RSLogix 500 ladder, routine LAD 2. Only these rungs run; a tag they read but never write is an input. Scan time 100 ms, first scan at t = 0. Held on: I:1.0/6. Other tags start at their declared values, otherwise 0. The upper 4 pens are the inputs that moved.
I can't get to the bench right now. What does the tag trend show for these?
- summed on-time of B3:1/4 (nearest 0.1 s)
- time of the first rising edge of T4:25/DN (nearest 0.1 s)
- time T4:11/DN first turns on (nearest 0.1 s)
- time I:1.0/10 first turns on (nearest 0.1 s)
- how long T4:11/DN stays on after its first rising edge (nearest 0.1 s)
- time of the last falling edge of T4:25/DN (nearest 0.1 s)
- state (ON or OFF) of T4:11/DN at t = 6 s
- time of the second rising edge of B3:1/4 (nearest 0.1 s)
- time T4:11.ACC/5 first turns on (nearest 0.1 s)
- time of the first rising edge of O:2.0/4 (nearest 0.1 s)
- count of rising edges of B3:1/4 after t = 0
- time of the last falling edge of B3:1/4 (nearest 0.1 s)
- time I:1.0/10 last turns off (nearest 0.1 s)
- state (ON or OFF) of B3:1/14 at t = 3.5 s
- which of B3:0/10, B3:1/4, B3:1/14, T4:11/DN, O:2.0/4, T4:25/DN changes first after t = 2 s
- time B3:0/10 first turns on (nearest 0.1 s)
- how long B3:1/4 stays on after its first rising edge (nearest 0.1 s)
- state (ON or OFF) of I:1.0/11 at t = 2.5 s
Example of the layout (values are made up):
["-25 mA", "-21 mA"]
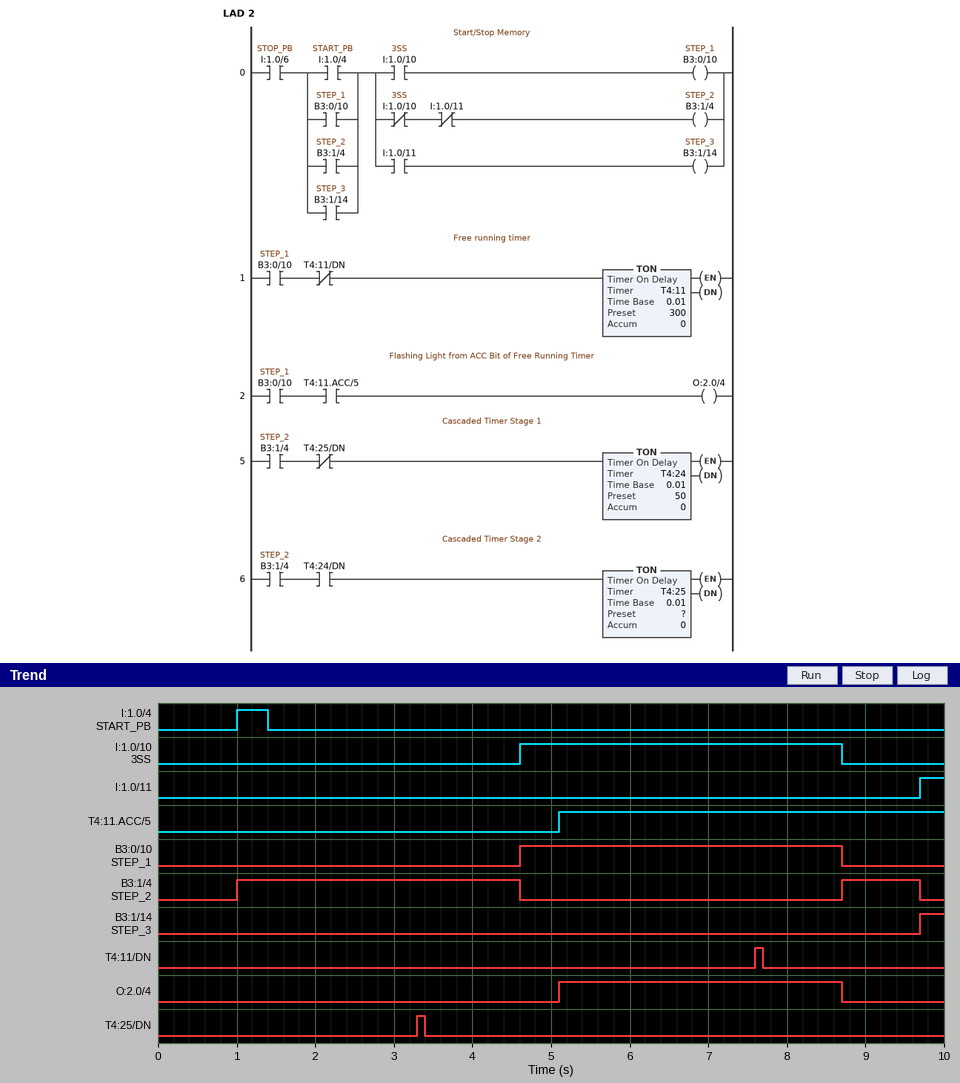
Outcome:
["4.6 s", "3.3 s", "7.6 s", "4.6 s", "0.1 s", "3.4 s", "OFF", "8.7 s", "5.1 s", "5.1 s", "2", "9.7 s", "8.7 s", "OFF", "T4:25/DN", "4.6 s", "3.6 s", "OFF"]
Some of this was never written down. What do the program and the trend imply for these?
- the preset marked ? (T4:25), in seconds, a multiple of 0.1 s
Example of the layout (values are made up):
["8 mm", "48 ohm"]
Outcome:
["1.8 s"]
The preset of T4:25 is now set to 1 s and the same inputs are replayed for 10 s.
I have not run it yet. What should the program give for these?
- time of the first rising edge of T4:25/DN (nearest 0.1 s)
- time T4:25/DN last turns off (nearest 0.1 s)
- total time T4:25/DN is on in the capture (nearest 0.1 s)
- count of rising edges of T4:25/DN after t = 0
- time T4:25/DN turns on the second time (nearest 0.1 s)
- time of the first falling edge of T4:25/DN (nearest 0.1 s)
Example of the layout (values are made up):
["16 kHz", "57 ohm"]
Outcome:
["2.5 s", "4.3 s", "0.2 s", "2", "4.2 s", "2.6 s"]
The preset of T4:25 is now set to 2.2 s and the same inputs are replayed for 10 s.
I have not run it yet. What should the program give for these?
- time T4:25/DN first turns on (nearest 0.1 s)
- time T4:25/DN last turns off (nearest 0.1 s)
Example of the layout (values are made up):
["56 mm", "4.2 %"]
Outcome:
["3.7 s", "3.8 s"]
